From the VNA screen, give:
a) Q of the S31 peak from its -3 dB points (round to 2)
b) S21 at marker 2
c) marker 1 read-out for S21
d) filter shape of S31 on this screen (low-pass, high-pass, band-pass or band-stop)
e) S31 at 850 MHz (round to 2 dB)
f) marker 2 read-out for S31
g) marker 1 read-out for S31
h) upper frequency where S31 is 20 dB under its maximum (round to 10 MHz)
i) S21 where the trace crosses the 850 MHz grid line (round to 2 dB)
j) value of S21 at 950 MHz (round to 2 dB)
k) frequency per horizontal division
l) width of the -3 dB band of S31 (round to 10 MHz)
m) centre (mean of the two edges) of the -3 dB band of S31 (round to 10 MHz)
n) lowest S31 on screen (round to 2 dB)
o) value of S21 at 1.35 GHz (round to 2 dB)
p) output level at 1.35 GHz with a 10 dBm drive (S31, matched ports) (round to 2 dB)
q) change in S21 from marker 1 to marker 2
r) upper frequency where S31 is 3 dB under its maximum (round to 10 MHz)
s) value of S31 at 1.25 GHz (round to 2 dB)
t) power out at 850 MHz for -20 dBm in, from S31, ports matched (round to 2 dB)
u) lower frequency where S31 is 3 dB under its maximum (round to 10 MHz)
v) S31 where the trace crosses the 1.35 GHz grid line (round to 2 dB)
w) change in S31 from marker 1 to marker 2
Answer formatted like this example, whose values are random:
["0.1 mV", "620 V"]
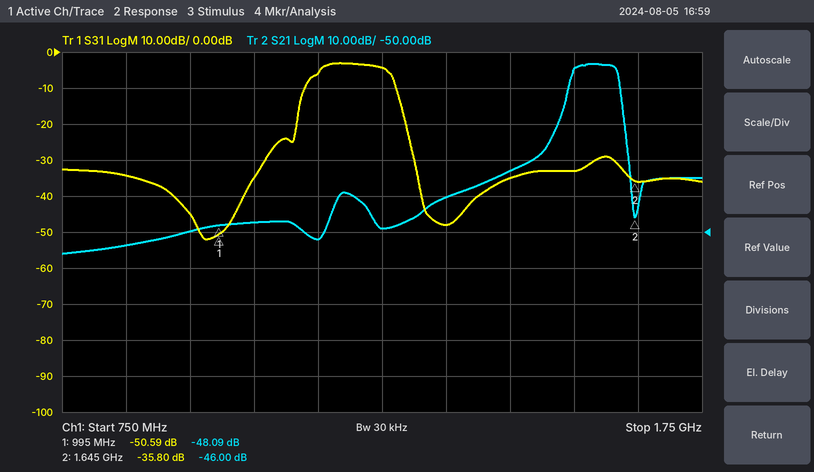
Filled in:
["10", "-46.00 dB", "-48.09 dB", "band-pass", "-34 dB", "-35.80 dB", "-50.59 dB", "1.29 GHz", "-54 dB", "-50 dB", "100 MHz", "110 MHz", "1.21 GHz", "-52 dB", "-40 dB", "-38 dBm", "2.09 dB", "1.26 GHz", "-4 dB", "-54 dBm", "1.15 GHz", "-48 dB", "14.79 dB"]
